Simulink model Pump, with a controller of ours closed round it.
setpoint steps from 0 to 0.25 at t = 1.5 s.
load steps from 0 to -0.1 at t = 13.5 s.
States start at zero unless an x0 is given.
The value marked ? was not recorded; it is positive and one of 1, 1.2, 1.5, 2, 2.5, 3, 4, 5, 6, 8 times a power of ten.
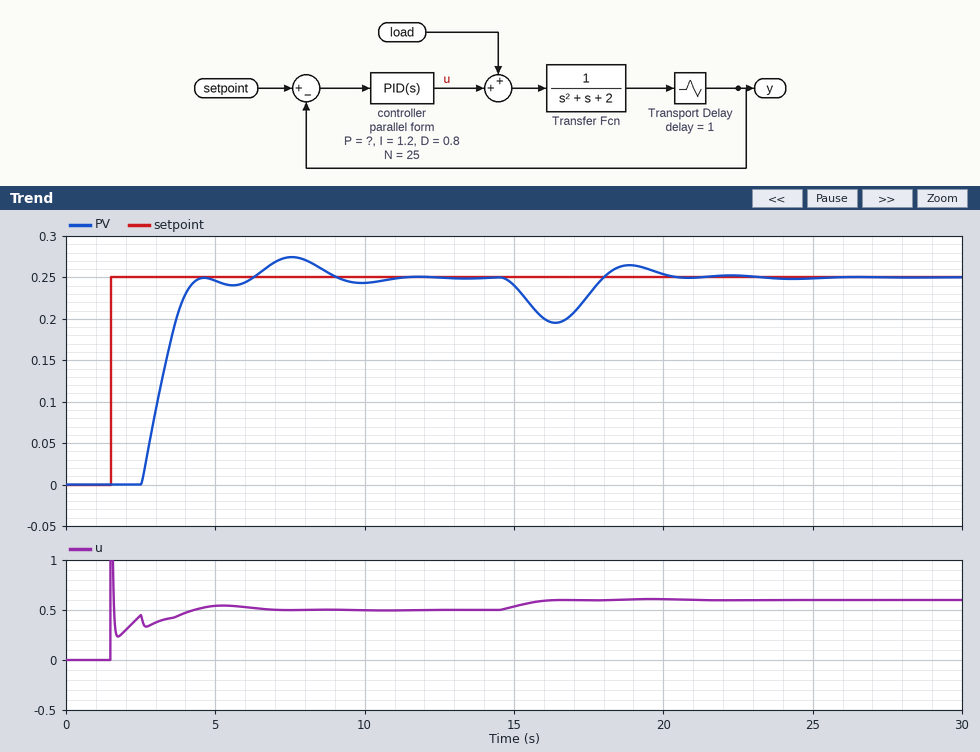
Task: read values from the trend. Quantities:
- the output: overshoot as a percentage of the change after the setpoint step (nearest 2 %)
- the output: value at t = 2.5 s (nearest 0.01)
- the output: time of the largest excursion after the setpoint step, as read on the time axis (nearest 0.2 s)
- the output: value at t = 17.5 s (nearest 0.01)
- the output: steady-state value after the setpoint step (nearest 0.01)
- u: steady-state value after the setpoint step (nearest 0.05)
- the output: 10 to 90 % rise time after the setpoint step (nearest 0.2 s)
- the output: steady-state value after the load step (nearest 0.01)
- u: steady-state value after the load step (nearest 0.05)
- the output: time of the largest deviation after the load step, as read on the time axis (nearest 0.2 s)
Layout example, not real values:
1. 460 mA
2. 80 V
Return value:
1. 10 %
2. 0.00
3. 7.6 s
4. 0.23
5. 0.25
6. 0.50
7. 1.2 s
8. 0.25
9. 0.60
10. 16.4 s
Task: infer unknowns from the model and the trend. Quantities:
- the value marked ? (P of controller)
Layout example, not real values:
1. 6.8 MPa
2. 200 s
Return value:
1. 0.6
